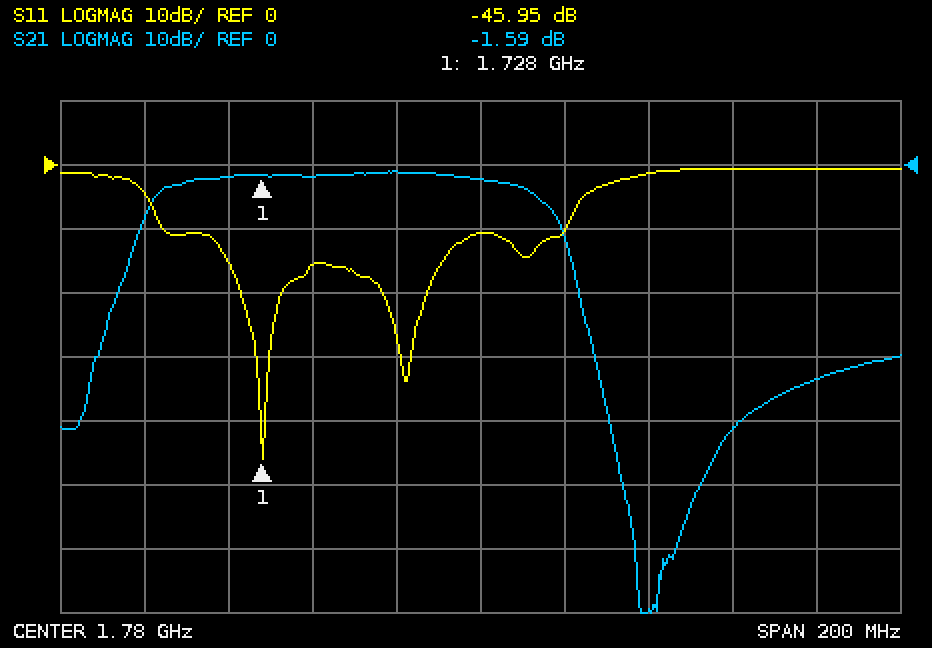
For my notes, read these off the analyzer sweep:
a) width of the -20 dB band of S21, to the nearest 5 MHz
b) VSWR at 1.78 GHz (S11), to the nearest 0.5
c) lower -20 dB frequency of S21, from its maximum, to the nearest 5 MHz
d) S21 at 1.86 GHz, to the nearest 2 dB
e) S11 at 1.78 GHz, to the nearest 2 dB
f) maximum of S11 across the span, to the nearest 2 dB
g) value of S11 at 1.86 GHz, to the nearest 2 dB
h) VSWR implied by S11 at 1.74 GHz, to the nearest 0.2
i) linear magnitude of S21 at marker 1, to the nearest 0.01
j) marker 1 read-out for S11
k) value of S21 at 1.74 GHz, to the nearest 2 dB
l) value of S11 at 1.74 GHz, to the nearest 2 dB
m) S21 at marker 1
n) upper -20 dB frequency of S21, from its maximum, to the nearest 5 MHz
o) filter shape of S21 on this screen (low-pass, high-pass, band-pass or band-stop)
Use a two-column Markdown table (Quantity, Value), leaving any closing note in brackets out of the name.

| Quantity | Value |
|---|---|
| width of the -20 dB band of S21, to the nearest 5 MHz | 110 MHz |
| VSWR at 1.78 GHz (S11), to the nearest 0.5 | 2.0 |
| lower -20 dB frequency of S21, from its maximum, to the nearest 5 MHz | 1.695 GHz |
| S21 at 1.86 GHz, to the nearest 2 dB | -34 dB |
| S11 at 1.78 GHz, to the nearest 2 dB | -10 dB |
| maximum of S11 across the span, to the nearest 2 dB | 0 dB |
| value of S11 at 1.86 GHz, to the nearest 2 dB | 0 dB |
| VSWR implied by S11 at 1.74 GHz, to the nearest 0.2 | 1.4 |
| linear magnitude of S21 at marker 1, to the nearest 0.01 | 0.83 |
| marker 1 read-out for S11 | -45.95 dB |
| value of S21 at 1.74 GHz, to the nearest 2 dB | -2 dB |
| value of S11 at 1.74 GHz, to the nearest 2 dB | -16 dB |
| S21 at marker 1 | -1.59 dB |
| upper -20 dB frequency of S21, from its maximum, to the nearest 5 MHz | 1.805 GHz |
| filter shape of S21 on this screen | band-pass |
